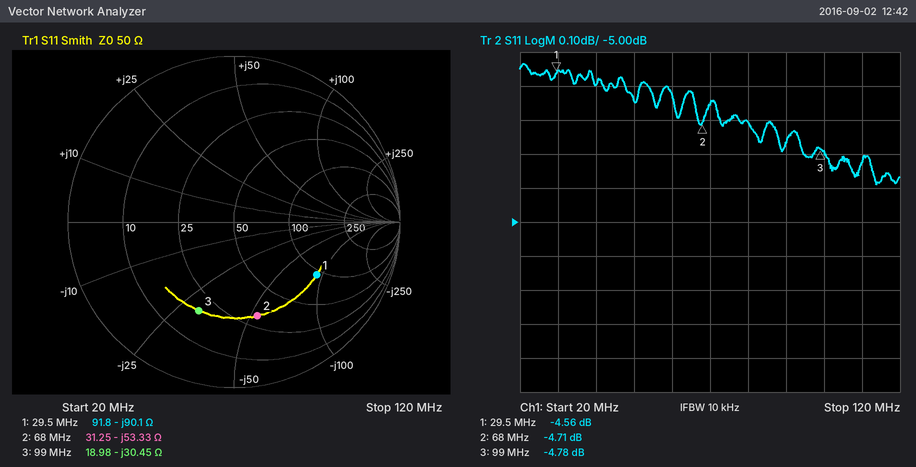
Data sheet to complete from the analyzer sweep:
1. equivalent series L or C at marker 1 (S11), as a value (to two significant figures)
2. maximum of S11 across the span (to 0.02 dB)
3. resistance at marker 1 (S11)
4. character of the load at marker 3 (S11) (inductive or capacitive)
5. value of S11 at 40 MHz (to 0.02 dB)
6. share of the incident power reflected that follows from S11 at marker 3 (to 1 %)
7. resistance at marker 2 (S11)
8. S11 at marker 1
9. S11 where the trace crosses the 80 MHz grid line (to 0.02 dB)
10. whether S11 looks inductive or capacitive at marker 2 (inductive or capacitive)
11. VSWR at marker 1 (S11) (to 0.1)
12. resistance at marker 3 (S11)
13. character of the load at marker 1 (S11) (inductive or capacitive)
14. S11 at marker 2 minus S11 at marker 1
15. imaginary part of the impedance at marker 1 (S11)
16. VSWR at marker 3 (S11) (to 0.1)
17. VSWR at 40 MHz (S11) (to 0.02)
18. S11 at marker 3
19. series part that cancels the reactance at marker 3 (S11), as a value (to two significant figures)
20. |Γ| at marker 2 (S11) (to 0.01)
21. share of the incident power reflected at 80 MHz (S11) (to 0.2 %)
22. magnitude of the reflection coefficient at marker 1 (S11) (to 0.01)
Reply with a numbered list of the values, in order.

1. 60 pF
2. -4.54 dB
3. 91.8 Ω
4. capacitive
5. -4.60 dB
6. 33 %
7. 31.25 Ω
8. -4.56 dB
9. -4.70 dB
10. capacitive
11. 3.9
12. 18.98 Ω
13. capacitive
14. -0.15 dB
15. -90.1 Ω
16. 3.7
17. 3.86
18. -4.78 dB
19. 49 nH
20. 0.58
21. 33.8 %
22. 0.59
